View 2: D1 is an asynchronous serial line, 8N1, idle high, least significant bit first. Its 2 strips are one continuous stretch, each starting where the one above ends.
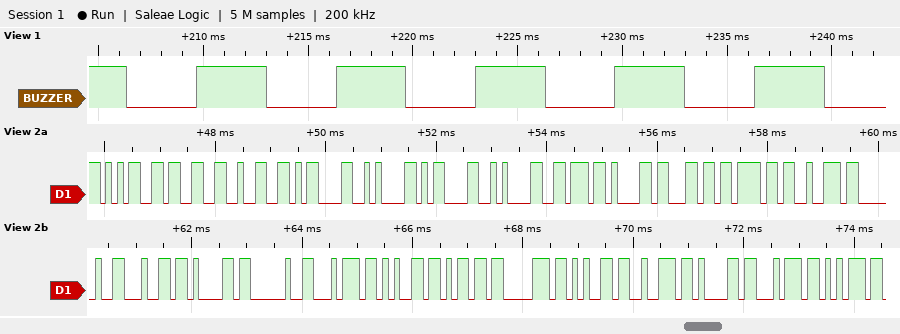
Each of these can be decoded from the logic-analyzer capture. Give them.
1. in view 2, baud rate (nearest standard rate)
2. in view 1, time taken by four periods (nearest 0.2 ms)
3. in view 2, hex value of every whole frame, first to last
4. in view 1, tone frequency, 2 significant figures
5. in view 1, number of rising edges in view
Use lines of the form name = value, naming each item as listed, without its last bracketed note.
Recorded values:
in view 2, baud rate = 9600 baud
in view 1, time taken by four periods = 26.6 ms
in view 2, hex value of every whole frame, first to last = 35 33 32 0D 0A 0D 0A 76 61 6C 6F 72 20 64 61 20 74 65 6D 70 65 72 61 74 75
in view 1, tone frequency, 2 significant figures = 150 Hz
in view 1, number of rising edges in view = 5
